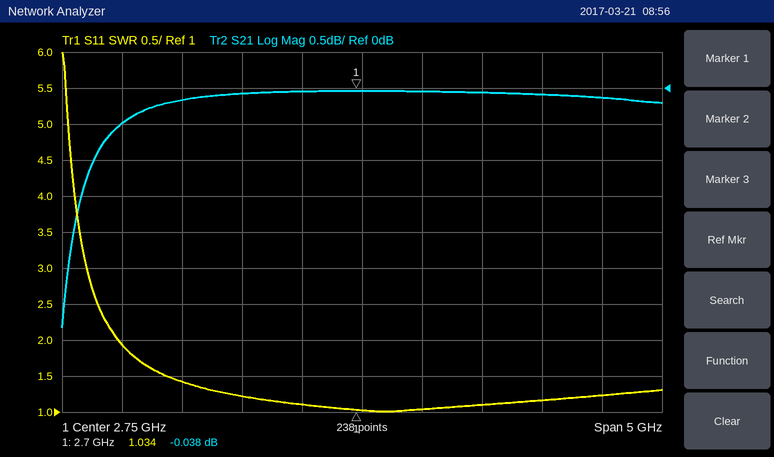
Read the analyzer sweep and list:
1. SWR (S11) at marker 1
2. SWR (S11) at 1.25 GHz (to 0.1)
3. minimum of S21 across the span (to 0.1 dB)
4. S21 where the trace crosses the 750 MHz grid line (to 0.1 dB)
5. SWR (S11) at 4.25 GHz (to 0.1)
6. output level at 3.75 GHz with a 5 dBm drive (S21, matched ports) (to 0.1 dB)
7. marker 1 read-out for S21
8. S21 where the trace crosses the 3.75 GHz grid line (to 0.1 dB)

1.034
1.4
-3.3 dB
-0.5 dB
1.2
4.9 dBm
-0.038 dB
-0.1 dB
